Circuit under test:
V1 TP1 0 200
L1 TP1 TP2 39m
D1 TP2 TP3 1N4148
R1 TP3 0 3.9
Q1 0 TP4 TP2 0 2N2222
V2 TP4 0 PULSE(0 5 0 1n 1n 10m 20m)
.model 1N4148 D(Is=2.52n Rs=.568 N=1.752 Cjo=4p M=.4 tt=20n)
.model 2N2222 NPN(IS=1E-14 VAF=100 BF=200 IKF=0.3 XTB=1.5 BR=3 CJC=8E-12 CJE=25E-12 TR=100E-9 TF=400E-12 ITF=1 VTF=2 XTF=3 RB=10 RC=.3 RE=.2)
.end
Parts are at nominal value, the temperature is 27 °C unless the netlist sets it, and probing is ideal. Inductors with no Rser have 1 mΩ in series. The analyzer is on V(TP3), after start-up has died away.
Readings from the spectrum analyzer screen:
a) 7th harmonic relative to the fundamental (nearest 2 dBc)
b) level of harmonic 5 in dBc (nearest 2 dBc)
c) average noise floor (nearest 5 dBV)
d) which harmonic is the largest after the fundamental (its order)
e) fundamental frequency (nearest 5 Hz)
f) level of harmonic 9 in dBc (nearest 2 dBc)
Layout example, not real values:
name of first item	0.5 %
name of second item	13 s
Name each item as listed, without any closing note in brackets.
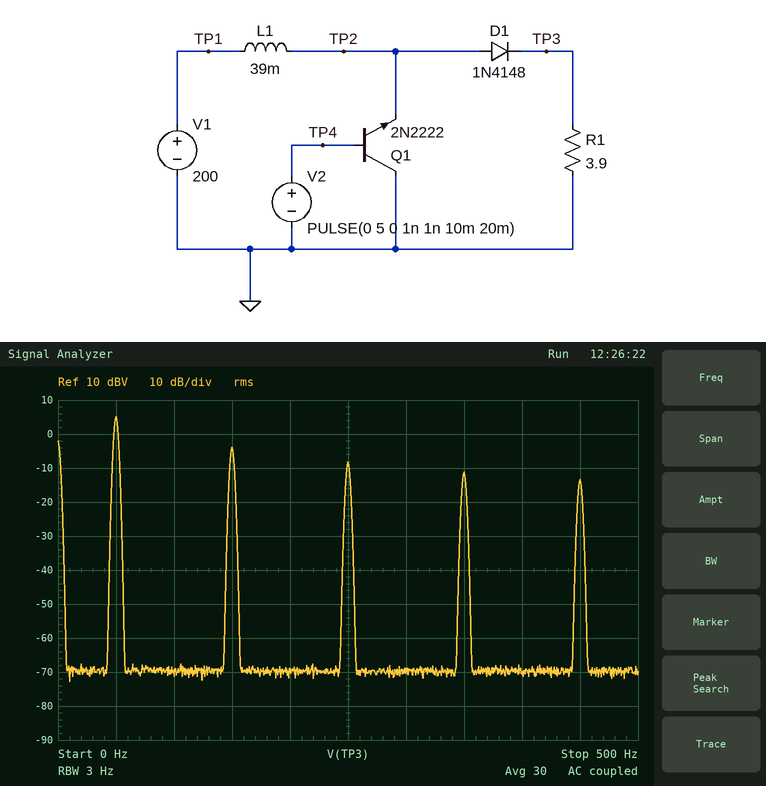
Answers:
7th harmonic relative to the fundamental	-16 dBc
level of harmonic 5 in dBc	-14 dBc
average noise floor	-70 dBV
which harmonic is the largest after the fundamental	3
fundamental frequency	50 Hz
level of harmonic 9 in dBc	-18 dBc
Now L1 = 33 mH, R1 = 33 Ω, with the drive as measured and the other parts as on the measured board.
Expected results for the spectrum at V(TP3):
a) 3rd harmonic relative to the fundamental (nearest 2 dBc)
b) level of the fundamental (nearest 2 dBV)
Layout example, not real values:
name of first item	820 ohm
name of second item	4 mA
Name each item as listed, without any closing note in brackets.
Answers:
3rd harmonic relative to the fundamental	-2 dBc
level of the fundamental	14 dBV
